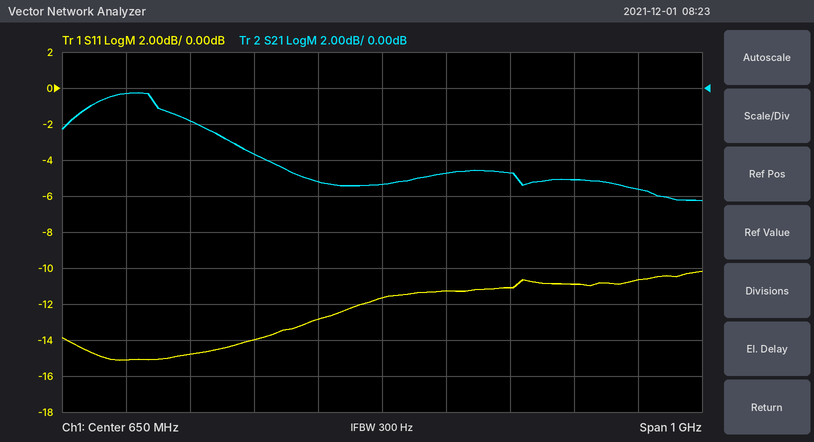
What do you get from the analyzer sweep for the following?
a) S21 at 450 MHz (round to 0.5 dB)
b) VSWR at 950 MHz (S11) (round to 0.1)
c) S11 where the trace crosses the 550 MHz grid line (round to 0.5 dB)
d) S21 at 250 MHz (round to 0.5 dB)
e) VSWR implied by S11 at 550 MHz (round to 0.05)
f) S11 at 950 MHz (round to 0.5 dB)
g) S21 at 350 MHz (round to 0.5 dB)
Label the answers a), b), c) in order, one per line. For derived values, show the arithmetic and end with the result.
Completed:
a) -3.5 dB
b) |Γ| = 10^(-11/20) = 0.2818; VSWR = (1 + 0.2818)/(1 − 0.2818) ≈ 1.8
c) -13.0 dB
d) -0.5 dB
e) |Γ| = 10^(-13/20) = 0.2239; VSWR = (1 + 0.2239)/(1 − 0.2239) ≈ 1.58, so 1.60 to the nearest 0.05
f) -11.0 dB
g) -2.0 dB
